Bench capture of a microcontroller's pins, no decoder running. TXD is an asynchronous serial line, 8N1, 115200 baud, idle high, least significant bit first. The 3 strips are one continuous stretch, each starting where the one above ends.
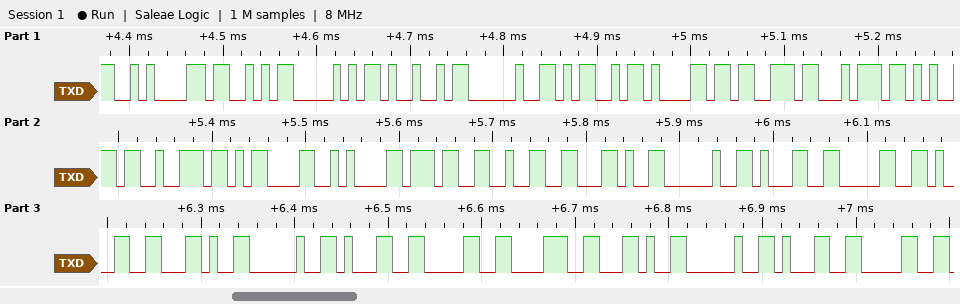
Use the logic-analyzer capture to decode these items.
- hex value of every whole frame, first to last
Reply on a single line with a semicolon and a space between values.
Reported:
0A 53 50 49 20 4D 61 73 74 65 72 0D 0A 37 32 2C 20 31 30 31 2C 20 31 30 38 2C 20 31 30
